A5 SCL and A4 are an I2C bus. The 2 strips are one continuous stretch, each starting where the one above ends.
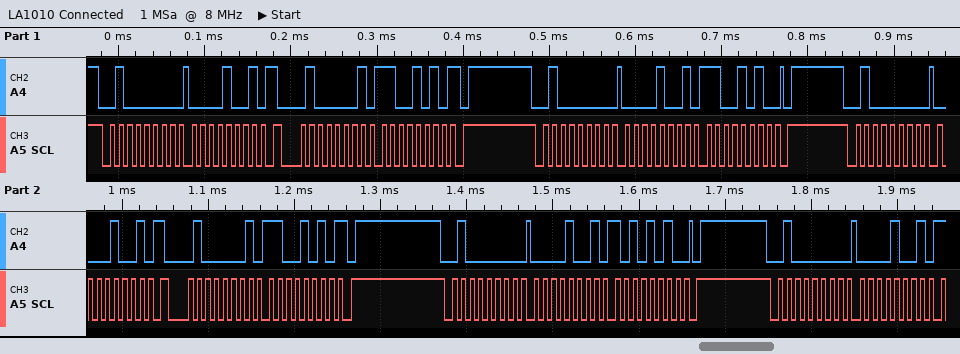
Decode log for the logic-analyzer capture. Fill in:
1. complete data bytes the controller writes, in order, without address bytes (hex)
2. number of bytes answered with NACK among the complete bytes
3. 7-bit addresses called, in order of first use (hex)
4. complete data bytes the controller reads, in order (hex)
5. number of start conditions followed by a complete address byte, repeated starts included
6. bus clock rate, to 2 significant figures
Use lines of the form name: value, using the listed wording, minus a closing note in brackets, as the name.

complete data bytes the controller writes, in order, without address bytes: 09 09 CA 09 09 AA 09
number of bytes answered with NACK among the complete bytes: 2
7-bit addresses called, in order of first use: 0x20
complete data bytes the controller reads, in order: CA CA
number of start conditions followed by a complete address byte, repeated starts included: 7
bus clock rate, to 2 significant figures: 100 kHz
